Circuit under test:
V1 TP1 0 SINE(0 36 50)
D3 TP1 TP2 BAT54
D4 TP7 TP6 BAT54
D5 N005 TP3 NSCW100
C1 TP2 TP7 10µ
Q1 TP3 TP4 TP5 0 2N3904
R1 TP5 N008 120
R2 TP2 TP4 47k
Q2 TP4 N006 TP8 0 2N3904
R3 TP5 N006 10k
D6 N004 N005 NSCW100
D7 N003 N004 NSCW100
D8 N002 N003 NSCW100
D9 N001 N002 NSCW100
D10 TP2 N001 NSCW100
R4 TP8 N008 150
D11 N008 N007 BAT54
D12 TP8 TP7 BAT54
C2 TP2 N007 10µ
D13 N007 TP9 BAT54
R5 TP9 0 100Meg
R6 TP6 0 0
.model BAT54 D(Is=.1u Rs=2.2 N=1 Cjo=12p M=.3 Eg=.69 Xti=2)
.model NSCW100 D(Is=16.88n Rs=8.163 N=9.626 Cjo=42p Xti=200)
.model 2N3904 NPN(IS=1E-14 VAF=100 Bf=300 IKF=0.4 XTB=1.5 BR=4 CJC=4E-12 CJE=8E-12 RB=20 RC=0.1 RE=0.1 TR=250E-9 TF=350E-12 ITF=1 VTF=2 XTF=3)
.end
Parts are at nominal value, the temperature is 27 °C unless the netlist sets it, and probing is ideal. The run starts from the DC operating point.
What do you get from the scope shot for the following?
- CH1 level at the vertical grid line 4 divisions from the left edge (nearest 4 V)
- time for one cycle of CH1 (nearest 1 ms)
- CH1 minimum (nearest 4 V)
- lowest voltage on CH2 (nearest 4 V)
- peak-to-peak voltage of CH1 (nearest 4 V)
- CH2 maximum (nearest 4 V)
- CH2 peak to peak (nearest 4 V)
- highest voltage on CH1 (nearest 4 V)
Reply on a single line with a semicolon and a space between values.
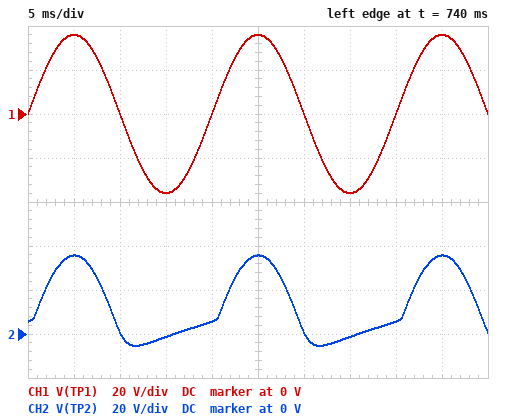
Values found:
0 V; 20 ms; -36 V; -4 V; 72 V; 36 V; 40 V; 36 V
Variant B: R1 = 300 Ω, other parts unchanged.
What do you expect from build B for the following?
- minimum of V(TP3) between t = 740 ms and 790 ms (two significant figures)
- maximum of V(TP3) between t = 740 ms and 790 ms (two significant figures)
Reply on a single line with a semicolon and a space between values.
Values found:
-22 V; 19 V
